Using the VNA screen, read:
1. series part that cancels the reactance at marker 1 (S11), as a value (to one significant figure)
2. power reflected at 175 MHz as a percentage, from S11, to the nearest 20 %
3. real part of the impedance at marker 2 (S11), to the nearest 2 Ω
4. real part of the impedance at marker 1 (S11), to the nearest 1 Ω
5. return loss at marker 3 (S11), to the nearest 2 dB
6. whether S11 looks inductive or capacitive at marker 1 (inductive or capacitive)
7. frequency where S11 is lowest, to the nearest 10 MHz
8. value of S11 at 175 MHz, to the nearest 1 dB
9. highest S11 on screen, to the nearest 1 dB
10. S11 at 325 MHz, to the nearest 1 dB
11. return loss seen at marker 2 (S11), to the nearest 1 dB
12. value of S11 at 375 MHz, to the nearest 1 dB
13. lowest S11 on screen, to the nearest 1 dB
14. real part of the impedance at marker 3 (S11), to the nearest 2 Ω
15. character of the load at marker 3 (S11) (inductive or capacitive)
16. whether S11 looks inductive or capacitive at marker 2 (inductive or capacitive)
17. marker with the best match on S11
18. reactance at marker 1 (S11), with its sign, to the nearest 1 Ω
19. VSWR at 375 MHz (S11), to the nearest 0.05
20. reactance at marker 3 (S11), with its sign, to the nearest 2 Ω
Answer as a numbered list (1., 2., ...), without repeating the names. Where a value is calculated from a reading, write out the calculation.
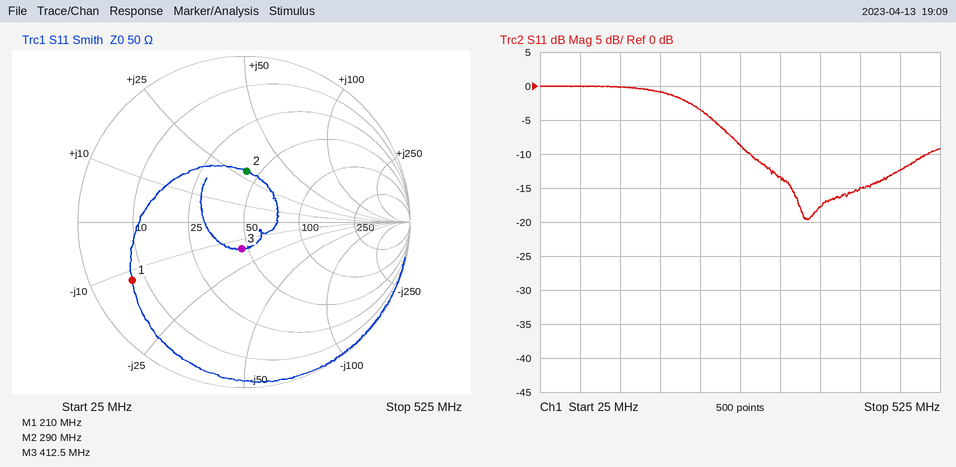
1. L = 12 Ω/(2π × 210 MHz) ≈ 9 nH
2. 10^(-1/10) ≈ 79.4 %, so 80 % to the nearest 20 %
3. 42 Ω
4. 7 Ω
5. 16 dB
6. capacitive
7. 360 MHz
8. -1 dB
9. 0 dB
10. -13 dB
11. 10 dB
12. -18 dB
13. -20 dB
14. 46 Ω
15. capacitive
16. inductive
17. marker 3
18. -12 Ω
19. |Γ| = 10^(-18/20) = 0.1259; VSWR = (1 + 0.1259)/(1 − 0.1259) ≈ 1.29, so 1.30 to the nearest 0.05
20. -16 Ω
